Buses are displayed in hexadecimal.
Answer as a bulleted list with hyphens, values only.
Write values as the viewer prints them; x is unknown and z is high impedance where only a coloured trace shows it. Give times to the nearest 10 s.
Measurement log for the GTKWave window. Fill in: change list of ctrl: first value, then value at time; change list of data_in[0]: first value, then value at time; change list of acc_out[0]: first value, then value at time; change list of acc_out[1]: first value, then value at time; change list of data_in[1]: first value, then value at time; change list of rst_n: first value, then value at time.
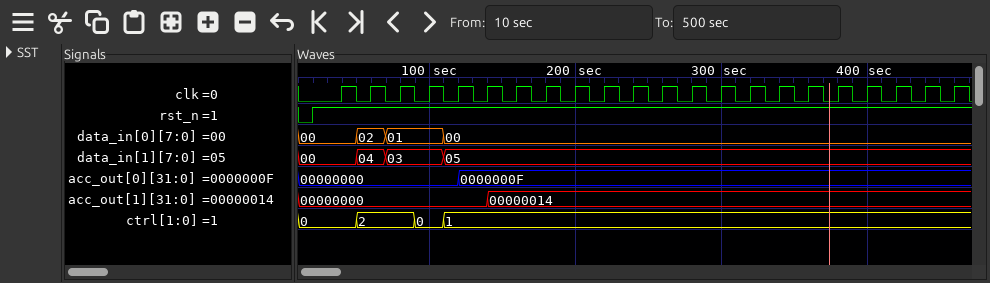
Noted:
- 0, 2 at 50 s, 0 at 90 s, 1 at 110 s
- 00, 02 at 50 s, 01 at 70 s, 00 at 110 s
- 00000000, 0000000F at 120 s
- 00000000, 00000014 at 140 s
- 00, 04 at 50 s, 03 at 70 s, 05 at 110 s
- 0, 1 at 20 s
